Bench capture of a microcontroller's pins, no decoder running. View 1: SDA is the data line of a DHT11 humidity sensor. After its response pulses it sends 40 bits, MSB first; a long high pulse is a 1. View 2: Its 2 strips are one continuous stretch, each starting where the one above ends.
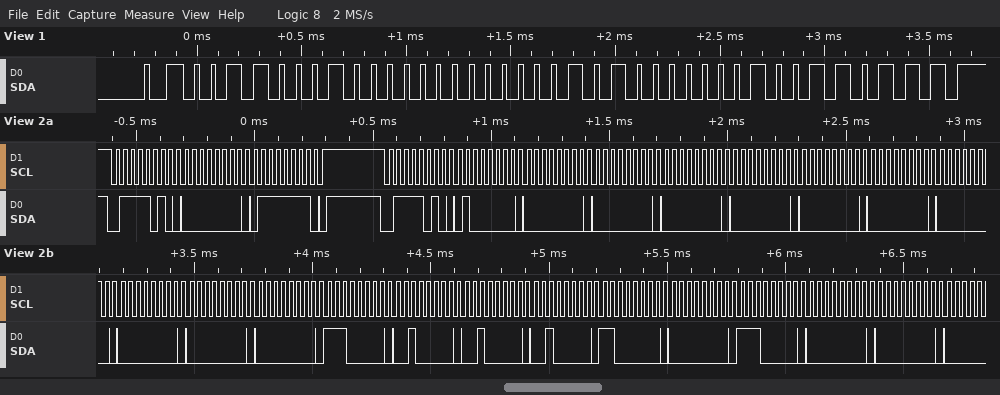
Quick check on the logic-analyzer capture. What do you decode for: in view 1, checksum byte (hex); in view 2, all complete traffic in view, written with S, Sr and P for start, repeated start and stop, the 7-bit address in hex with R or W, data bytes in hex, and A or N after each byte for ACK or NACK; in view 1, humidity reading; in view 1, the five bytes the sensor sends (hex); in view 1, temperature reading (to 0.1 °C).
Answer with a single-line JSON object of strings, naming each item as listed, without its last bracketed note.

{"in view 1, checksum byte": "0x37", "in view 2, all complete traffic in view, written with S, Sr and P for start, repeated start and stop, the 7-bit address in hex with R or W, data bytes in hex, and A or N after each byte for ACK or NACK": "S 3DW A 00 A 7F A P S 3DW A 40 A 00 A 00 A 00 A 00 A 00 A 00 A 00 A 00 A 00 A 00 A E0 A 20 A 20 A 20 A C0 A 00 A E0 A 00 A 00 A", "in view 1, humidity reading": "49 %", "in view 1, the five bytes the sensor sends": "31 00 05 01 37", "in view 1, temperature reading": "5.1 °C"}
